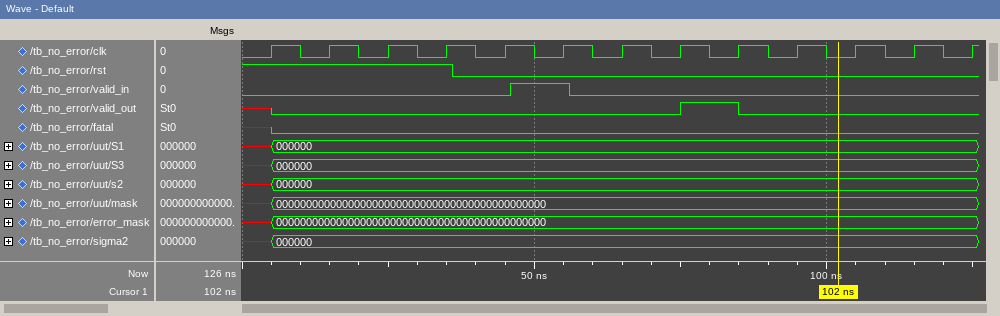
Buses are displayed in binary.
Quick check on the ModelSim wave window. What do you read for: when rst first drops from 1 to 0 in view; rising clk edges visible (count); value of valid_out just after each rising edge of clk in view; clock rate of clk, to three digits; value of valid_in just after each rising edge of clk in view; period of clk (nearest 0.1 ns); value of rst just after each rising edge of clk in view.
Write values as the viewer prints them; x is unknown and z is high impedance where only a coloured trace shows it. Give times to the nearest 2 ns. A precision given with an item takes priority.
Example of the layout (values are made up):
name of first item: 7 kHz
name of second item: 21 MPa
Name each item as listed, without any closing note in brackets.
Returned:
when rst first drops from 1 to 0 in view: 36 ns
rising clk edges visible: 13
value of valid_out just after each rising edge of clk in view: 0 0 0 0 0 0 0 1 0 0 0 0 0
clock rate of clk, to three digits: 100 MHz
value of valid_in just after each rising edge of clk in view: 0 0 0 0 0 1 0 0 0 0 0 0 0
period of clk: 10 ns
value of rst just after each rising edge of clk in view: 1 1 1 1 0 0 0 0 0 0 0 0 0
